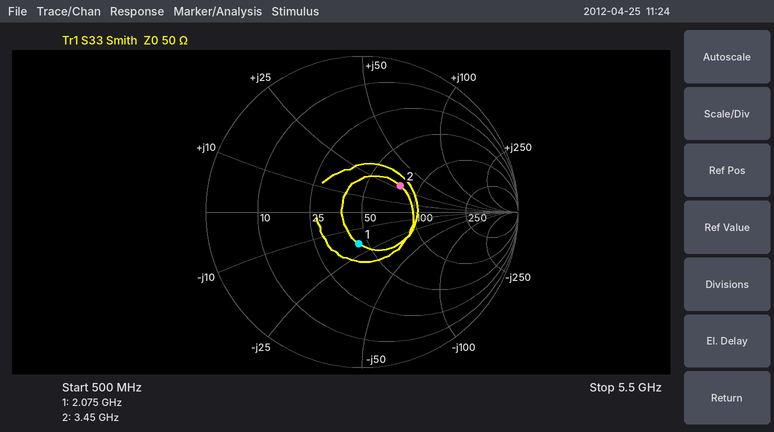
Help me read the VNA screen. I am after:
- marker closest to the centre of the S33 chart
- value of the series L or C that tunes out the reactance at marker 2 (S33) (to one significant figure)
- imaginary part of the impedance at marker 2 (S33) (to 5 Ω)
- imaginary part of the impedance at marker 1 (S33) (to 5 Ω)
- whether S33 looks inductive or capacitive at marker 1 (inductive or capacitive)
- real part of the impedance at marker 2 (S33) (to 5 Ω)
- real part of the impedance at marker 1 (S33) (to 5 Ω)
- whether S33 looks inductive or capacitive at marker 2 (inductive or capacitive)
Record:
marker 1
2 pF
+30 Ω
-20 Ω
capacitive
75 Ω
45 Ω
inductive
